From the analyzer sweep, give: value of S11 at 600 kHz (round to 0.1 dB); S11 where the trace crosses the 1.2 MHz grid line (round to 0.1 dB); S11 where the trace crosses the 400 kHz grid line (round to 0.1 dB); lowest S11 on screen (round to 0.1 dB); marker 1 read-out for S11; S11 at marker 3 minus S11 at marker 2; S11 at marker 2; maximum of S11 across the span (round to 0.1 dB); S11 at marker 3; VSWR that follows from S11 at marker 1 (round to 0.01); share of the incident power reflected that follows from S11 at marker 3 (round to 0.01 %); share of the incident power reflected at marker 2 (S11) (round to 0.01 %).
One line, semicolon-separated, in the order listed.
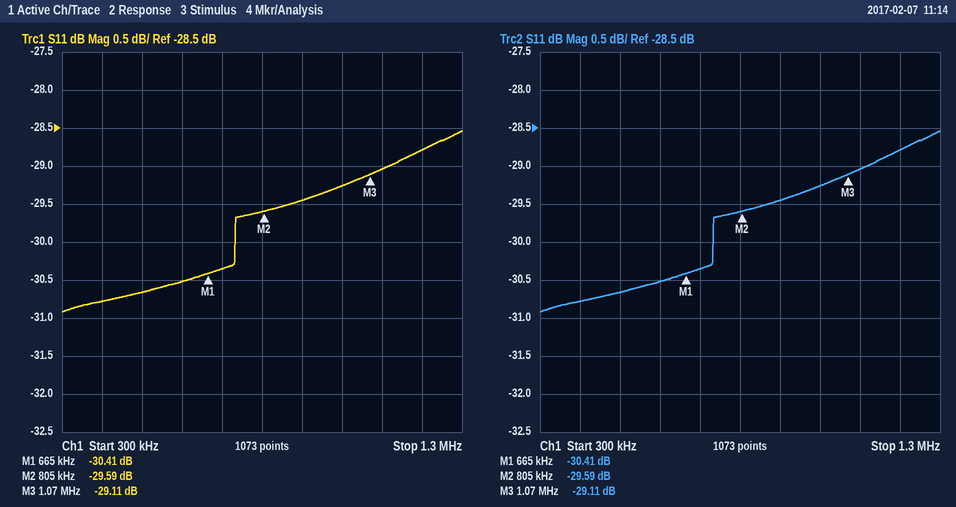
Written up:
-30.5 dB; -28.8 dB; -30.8 dB; -30.9 dB; -30.41 dB; 0.48 dB; -29.59 dB; -28.5 dB; -29.11 dB; 1.06; 0.12 %; 0.11 %
